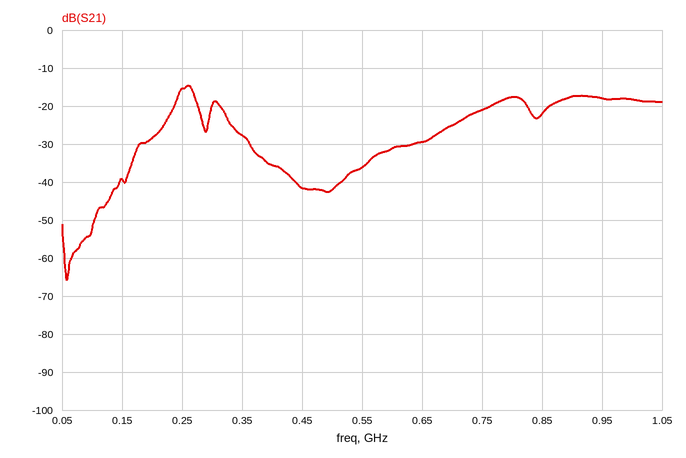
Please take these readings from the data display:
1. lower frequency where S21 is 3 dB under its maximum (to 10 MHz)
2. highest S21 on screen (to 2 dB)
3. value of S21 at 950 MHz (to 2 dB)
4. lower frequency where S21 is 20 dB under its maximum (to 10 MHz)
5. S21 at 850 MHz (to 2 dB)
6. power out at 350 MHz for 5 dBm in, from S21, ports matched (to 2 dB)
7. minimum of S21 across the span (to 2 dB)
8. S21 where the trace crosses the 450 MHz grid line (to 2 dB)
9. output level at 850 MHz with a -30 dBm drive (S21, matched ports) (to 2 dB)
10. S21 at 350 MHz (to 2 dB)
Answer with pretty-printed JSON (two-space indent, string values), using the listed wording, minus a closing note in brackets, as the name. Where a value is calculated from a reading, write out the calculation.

{
  "lower frequency where S21 is 3 dB under its maximum": "240 MHz",
  "highest S21 on screen": "-14 dB",
  "value of S21 at 950 MHz": "-18 dB",
  "lower frequency where S21 is 20 dB under its maximum": "170 MHz",
  "S21 at 850 MHz": "-22 dB",
  "power out at 350 MHz for 5 dBm in, from S21, ports matched": "5 dBm + (-28 dB) = -22 dBm",
  "minimum of S21 across the span": "-66 dB",
  "S21 where the trace crosses the 450 MHz grid line": "-42 dB",
  "output level at 850 MHz with a -30 dBm drive (S21, matched ports)": "-30 dBm + (-22 dB) = -52 dBm",
  "S21 at 350 MHz": "-28 dB"
}
